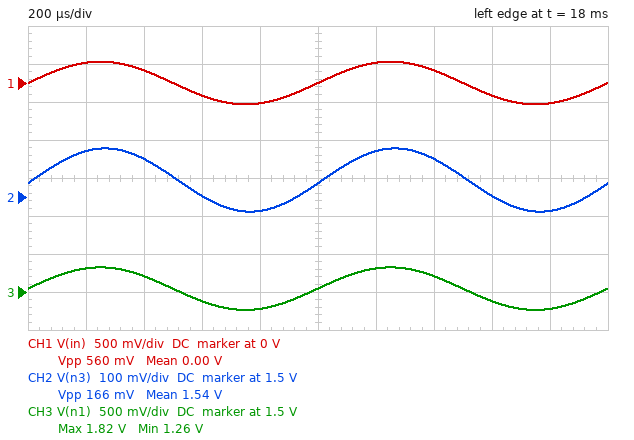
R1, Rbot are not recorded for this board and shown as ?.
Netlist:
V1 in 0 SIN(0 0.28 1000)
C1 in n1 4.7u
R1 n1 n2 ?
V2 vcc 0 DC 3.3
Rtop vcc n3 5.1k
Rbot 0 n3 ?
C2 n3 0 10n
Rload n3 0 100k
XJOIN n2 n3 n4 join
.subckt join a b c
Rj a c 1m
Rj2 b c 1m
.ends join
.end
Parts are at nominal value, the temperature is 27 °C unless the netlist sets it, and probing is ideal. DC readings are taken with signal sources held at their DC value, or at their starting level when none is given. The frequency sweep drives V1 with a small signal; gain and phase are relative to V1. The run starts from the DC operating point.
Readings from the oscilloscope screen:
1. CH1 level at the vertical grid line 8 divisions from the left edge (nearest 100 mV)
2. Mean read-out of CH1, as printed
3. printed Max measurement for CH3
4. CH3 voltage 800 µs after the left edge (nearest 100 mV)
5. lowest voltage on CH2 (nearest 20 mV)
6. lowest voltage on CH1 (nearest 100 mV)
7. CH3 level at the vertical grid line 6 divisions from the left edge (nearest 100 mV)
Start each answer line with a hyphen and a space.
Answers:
- -200 mV
- 0.00 V
- 1.82 V
- 1.3 V
- 1.46 V
- -300 mV
- 1.8 V
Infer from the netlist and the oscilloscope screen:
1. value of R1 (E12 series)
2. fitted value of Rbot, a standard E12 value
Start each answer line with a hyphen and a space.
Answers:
- 5.6 kΩ
- 4.7 kΩ
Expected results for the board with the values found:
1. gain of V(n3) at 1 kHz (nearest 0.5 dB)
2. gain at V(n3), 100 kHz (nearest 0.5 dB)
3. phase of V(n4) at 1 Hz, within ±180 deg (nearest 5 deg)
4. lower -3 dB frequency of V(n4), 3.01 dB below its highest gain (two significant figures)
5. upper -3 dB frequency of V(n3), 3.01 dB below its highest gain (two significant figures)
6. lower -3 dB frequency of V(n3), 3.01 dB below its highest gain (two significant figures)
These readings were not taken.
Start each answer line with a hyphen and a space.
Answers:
- -10.5 dB
- -31.0 dB
- 75 deg
- 4.2 Hz
- 9.5 kHz
- 4.2 Hz
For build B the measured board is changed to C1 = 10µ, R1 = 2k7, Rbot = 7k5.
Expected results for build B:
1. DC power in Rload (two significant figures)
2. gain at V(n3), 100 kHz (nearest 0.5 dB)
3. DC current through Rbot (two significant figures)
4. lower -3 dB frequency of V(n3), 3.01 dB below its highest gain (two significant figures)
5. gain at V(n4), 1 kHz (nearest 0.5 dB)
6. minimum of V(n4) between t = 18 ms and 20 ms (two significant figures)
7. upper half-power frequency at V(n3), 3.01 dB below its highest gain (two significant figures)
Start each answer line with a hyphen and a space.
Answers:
- 36 µW
- -24.5 dB
- 250 µA
- 2.8 Hz
- -5.5 dB
- 1.8 V
- 11 kHz
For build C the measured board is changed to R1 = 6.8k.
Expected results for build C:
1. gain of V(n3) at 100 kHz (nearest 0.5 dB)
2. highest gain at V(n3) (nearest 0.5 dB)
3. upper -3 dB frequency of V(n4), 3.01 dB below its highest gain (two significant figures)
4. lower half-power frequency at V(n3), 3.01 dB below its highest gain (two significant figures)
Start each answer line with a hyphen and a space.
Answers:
- -32.5 dB
- -11.5 dB
- 9.0 kHz
- 3.7 Hz
